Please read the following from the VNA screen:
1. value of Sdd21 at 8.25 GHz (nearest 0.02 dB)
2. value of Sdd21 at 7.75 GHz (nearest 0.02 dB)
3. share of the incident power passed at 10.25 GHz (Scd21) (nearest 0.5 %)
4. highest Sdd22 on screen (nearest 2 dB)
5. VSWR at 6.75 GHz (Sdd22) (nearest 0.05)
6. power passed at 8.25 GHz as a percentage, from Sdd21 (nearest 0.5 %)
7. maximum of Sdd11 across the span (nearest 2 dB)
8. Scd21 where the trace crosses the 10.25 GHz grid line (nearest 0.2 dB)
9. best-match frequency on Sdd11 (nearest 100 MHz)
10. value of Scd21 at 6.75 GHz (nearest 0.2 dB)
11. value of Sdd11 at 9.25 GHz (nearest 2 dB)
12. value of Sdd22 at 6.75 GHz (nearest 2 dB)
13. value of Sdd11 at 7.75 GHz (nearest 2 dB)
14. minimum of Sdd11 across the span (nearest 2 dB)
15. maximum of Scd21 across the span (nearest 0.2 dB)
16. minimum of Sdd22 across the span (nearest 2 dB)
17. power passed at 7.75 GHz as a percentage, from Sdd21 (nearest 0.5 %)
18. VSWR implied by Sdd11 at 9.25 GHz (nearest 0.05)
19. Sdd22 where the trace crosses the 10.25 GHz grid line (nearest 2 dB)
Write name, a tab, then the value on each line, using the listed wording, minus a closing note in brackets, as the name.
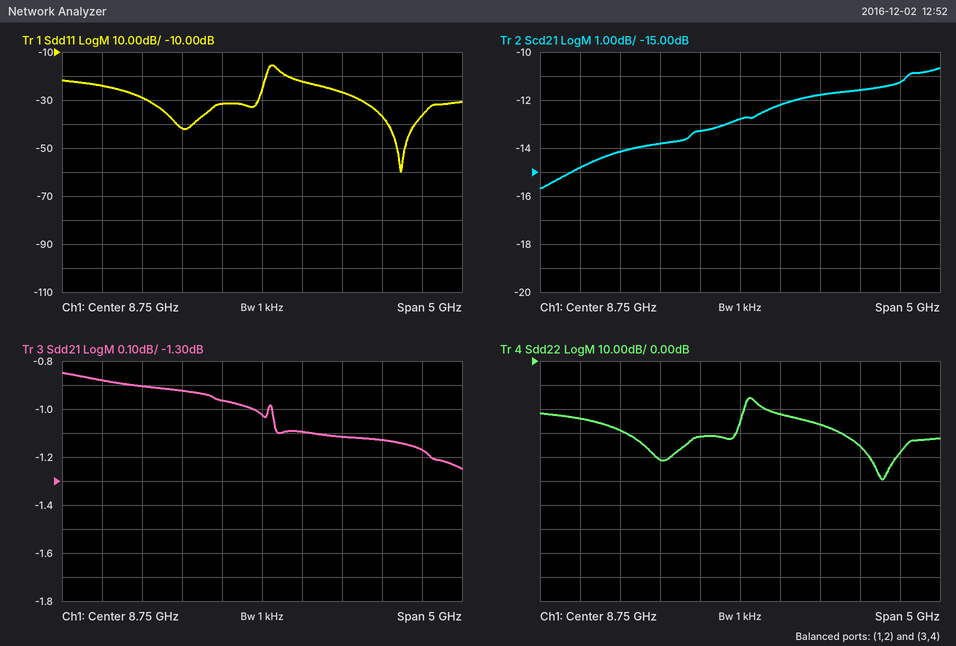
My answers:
value of Sdd21 at 8.25 GHz	-0.96 dB
value of Sdd21 at 7.75 GHz	-0.92 dB
share of the incident power passed at 10.25 GHz (Scd21)	7.0 %
highest Sdd22 on screen	-16 dB
VSWR at 6.75 GHz (Sdd22)	1.15
power passed at 8.25 GHz as a percentage, from Sdd21	80.0 %
maximum of Sdd11 across the span	-16 dB
Scd21 where the trace crosses the 10.25 GHz grid line	-11.6 dB
best-match frequency on Sdd11	10.5 GHz
value of Scd21 at 6.75 GHz	-14.8 dB
value of Sdd11 at 9.25 GHz	-22 dB
value of Sdd22 at 6.75 GHz	-24 dB
value of Sdd11 at 7.75 GHz	-42 dB
minimum of Sdd11 across the span	-60 dB
maximum of Scd21 across the span	-10.6 dB
minimum of Sdd22 across the span	-50 dB
power passed at 7.75 GHz as a percentage, from Sdd21	81.0 %
VSWR implied by Sdd11 at 9.25 GHz	1.15
Sdd22 where the trace crosses the 10.25 GHz grid line	-36 dB
